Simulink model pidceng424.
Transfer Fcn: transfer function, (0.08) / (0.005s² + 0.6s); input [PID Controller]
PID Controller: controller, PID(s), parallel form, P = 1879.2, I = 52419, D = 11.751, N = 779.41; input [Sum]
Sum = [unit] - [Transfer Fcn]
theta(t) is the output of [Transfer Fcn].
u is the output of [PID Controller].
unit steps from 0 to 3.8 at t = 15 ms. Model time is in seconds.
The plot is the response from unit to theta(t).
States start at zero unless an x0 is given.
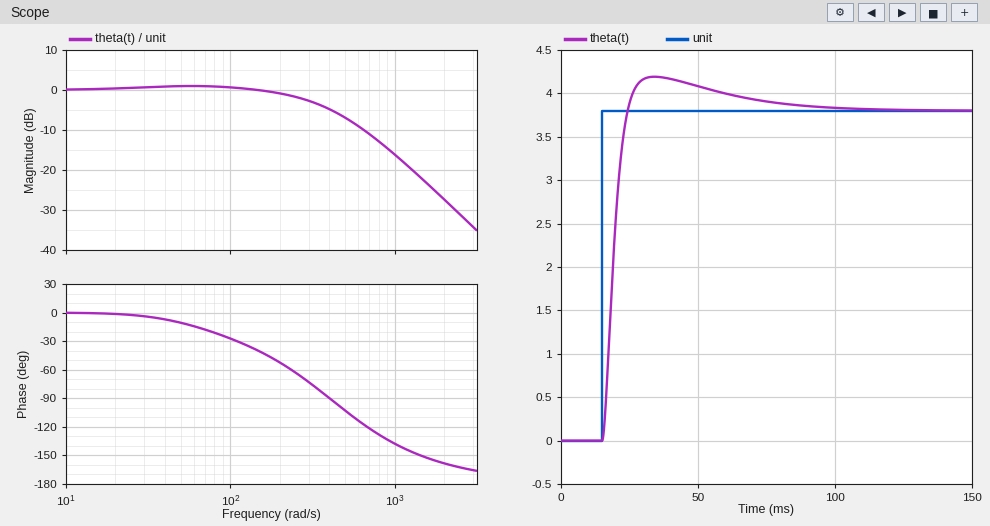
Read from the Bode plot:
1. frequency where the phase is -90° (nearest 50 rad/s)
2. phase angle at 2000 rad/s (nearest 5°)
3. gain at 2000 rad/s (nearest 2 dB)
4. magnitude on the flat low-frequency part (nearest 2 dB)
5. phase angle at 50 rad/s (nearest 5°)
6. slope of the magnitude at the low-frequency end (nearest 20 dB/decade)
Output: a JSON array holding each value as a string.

["400 rad/s", "-160°", "-28 dB", "0 dB", "-10°", "0 dB/decade"]
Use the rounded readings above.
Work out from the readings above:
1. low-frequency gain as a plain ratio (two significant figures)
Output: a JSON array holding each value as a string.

["1.0"]
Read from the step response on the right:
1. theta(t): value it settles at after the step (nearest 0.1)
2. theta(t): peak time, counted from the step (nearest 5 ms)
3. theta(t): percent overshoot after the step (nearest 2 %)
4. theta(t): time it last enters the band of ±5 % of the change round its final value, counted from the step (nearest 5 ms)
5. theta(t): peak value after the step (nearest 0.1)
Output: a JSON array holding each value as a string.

["3.8", "20 ms", "10 %", "45 ms", "4.2"]
